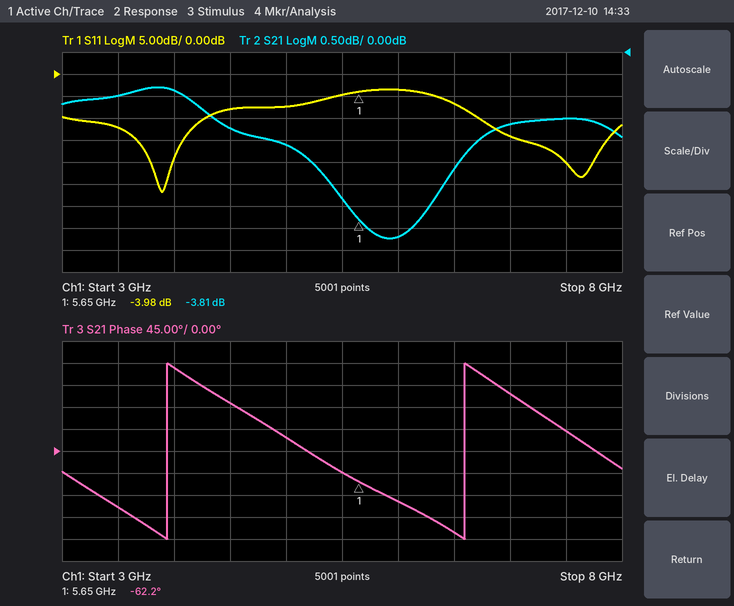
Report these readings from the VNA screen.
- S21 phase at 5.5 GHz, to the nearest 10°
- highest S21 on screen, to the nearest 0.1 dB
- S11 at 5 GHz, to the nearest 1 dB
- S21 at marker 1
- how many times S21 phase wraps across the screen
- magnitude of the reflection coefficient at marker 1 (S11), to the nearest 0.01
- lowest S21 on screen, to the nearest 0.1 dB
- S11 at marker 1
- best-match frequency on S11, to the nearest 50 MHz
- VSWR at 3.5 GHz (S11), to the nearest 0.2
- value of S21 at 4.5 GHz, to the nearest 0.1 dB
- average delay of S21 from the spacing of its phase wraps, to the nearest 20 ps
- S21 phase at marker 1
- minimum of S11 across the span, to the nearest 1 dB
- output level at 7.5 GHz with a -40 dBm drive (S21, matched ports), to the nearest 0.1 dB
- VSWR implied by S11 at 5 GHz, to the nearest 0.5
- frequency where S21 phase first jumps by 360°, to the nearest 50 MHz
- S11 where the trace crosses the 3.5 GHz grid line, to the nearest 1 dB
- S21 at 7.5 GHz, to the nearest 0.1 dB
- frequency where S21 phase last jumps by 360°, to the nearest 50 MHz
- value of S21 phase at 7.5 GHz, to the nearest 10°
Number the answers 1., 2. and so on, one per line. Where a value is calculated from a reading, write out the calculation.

1. -40°
2. -0.8 dB
3. -7 dB
4. -3.81 dB
5. 2
6. 10^(-3.98/20) ≈ 0.63
7. -4.2 dB
8. -3.98 dB
9. 3.90 GHz
10. |Γ| = 10^(-12/20) = 0.2512; VSWR = (1 + 0.2512)/(1 − 0.2512) ≈ 1.67, so 1.6 to the nearest 0.2
11. -1.7 dB
12. 1 cycle / (6.60 GHz − 3.95 GHz) ≈ 377 ps, so 380 ps to the nearest 20 ps
13. -62.2°
14. -27 dB
15. -40 dBm + (-1.5 dB) = -41.5 dBm
16. |Γ| = 10^(-7/20) = 0.4467; VSWR = (1 + 0.4467)/(1 − 0.4467) ≈ 2.61, so 2.5 to the nearest 0.5
17. 3.95 GHz
18. -12 dB
19. -1.5 dB
20. 6.60 GHz
21. 40°
